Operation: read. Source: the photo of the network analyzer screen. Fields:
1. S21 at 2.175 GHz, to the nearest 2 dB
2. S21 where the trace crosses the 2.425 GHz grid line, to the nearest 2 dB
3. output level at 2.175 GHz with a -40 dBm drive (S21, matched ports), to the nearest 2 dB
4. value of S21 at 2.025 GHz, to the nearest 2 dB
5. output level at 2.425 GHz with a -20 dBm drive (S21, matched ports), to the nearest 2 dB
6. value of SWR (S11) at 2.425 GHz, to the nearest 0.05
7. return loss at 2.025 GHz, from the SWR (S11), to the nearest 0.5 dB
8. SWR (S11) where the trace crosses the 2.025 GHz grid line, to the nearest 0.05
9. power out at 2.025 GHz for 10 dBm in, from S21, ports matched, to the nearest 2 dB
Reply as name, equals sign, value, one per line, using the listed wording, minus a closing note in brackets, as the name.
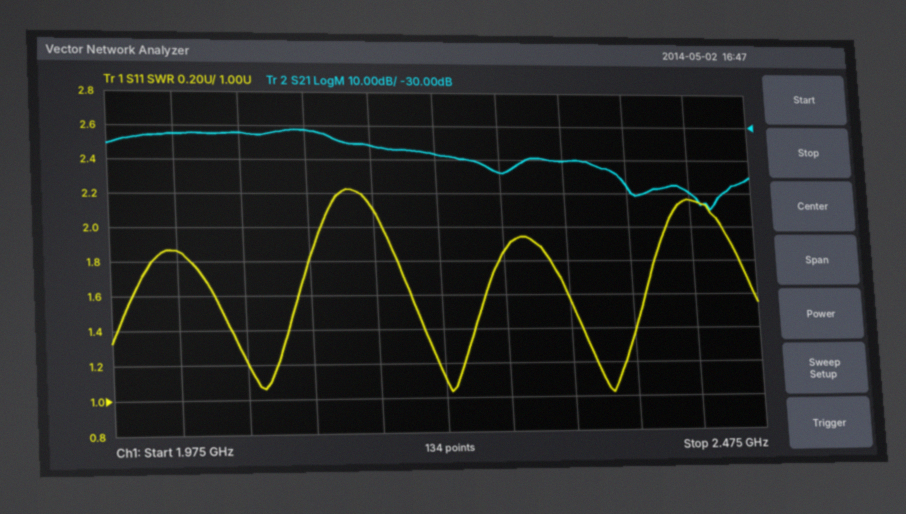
S21 at 2.175 GHz, to the nearest 2 dB = -36 dB
S21 where the trace crosses the 2.425 GHz grid line, to the nearest 2 dB = -50 dB
output level at 2.175 GHz with a -40 dBm drive (S21, matched ports), to the nearest 2 dB = -76 dBm
value of S21 at 2.025 GHz, to the nearest 2 dB = -32 dB
output level at 2.425 GHz with a -20 dBm drive (S21, matched ports), to the nearest 2 dB = -70 dBm
value of SWR (S11) at 2.425 GHz, to the nearest 0.05 = 2.15
return loss at 2.025 GHz, from the SWR (S11), to the nearest 0.5 dB = 10.5 dB
SWR (S11) where the trace crosses the 2.025 GHz grid line, to the nearest 0.05 = 1.85
power out at 2.025 GHz for 10 dBm in, from S21, ports matched, to the nearest 2 dB = -22 dBm
